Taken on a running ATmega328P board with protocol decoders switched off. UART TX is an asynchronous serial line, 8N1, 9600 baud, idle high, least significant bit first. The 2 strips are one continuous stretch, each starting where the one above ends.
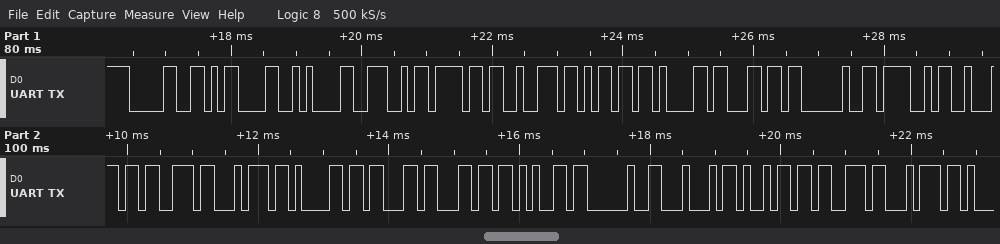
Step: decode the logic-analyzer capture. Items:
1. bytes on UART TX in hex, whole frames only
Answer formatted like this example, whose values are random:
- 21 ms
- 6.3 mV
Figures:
- 30 0D 0A 4E 6F 72 6D 61 6C 20 4F 62 73 74 61 63 6C 65 20 44 69 73 74
